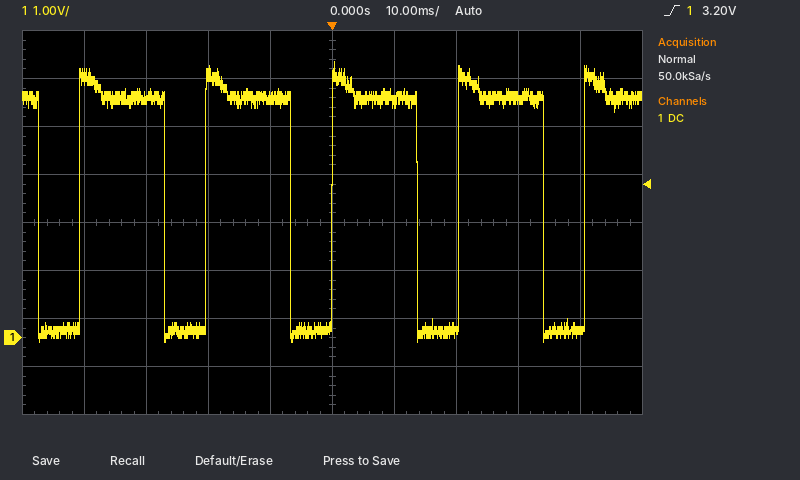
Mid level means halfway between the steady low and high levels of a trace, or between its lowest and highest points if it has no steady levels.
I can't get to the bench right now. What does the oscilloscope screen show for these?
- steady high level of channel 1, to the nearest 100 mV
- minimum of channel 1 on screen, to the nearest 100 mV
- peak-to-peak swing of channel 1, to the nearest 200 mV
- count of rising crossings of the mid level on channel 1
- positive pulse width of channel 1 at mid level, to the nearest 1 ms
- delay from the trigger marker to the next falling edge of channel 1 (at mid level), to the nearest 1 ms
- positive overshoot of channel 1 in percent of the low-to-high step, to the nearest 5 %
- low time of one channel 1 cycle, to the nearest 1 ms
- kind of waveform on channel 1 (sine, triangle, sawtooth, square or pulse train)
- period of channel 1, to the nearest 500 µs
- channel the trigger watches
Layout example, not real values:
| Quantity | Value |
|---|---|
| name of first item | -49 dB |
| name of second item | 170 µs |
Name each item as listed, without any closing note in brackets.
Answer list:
| Quantity | Value |
|---|---|
| steady high level of channel 1, to the nearest 100 mV | 5.0 V |
| minimum of channel 1 on screen, to the nearest 100 mV | -100 mV |
| peak-to-peak swing of channel 1, to the nearest 200 mV | 5.8 V |
| count of rising crossings of the mid level on channel 1 | 5 |
| positive pulse width of channel 1 at mid level, to the nearest 1 ms | 14 ms |
| delay from the trigger marker to the next falling edge of channel 1 (at mid level), to the nearest 1 ms | 14 ms |
| positive overshoot of channel 1 in percent of the low-to-high step, to the nearest 5 % | 15 % |
| low time of one channel 1 cycle, to the nearest 1 ms | 7 ms |
| kind of waveform on channel 1 | pulse train |
| period of channel 1, to the nearest 500 µs | 20.5 ms |
| channel the trigger watches | channel 1 |
